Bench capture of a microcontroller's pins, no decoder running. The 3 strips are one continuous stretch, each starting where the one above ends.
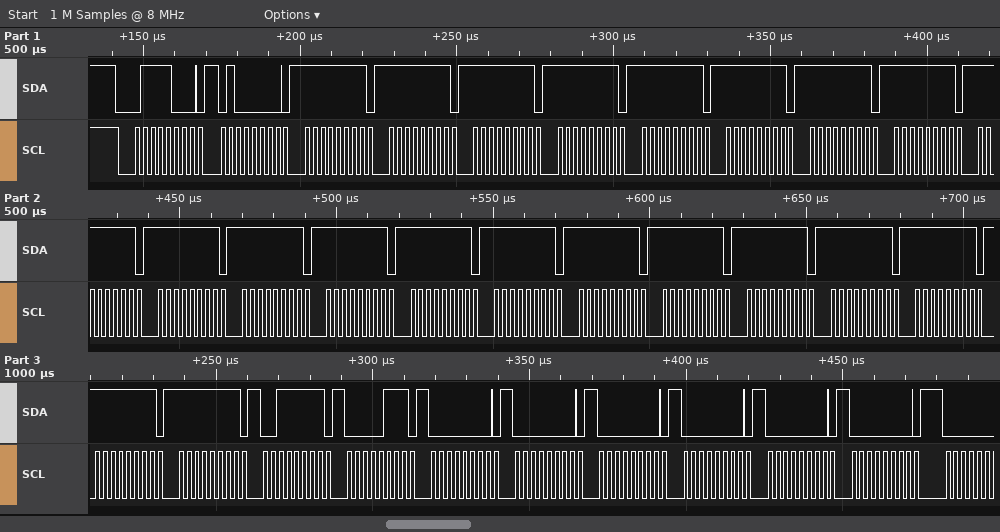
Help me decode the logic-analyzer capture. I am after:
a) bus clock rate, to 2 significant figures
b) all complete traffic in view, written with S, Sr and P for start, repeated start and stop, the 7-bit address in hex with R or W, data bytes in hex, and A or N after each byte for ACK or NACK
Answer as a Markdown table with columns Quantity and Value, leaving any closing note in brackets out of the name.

| Quantity | Value |
|---|---|
| bus clock rate, to 2 significant figures | 400 kHz |
| all complete traffic in view, written with S, Sr and P for start, repeated start and stop, the 7-bit address in hex with R or W, data bytes in hex, and A or N after each byte for ACK or NACK | S 3CW A 40 A FF A FF A FF A FF A FF A FF A FF A FF A FF A FF A FF A FF A FF A FF A FF A FF A FF A FF A FF A FF A FF A 3F A 07 A 00 A 00 A 00 A 00 A 00 A 00 A |
